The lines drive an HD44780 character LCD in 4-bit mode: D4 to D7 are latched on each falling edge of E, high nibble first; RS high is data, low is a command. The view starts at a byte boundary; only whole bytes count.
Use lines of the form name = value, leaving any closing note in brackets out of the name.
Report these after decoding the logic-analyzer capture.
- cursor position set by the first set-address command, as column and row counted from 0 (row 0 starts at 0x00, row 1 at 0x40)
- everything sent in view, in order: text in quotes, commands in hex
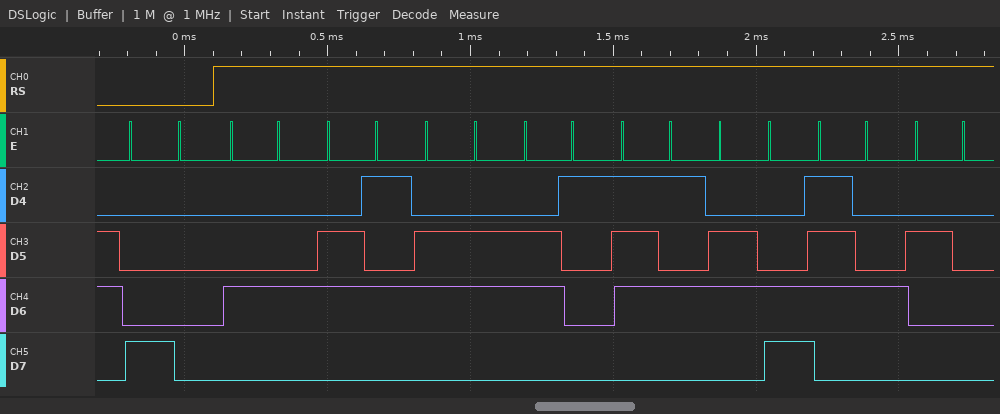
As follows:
cursor position set by the first set-address command, as column and row counted from 0 = column 0, row 0
everything sent in view, in order: text in quotes, commands in hex = 0x80 "Default "
